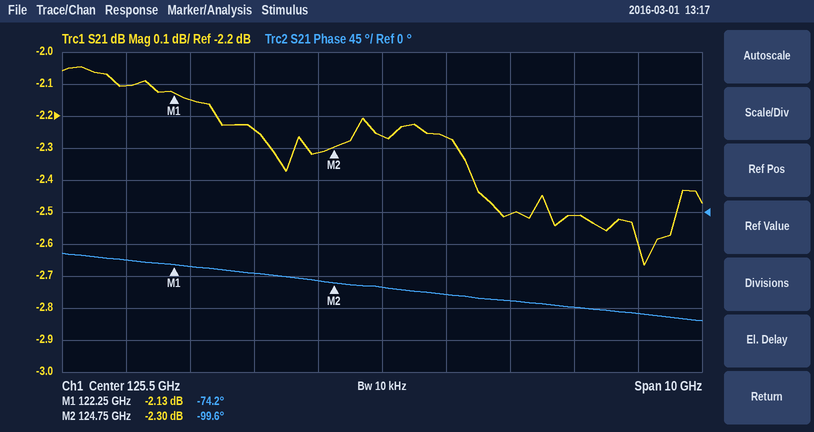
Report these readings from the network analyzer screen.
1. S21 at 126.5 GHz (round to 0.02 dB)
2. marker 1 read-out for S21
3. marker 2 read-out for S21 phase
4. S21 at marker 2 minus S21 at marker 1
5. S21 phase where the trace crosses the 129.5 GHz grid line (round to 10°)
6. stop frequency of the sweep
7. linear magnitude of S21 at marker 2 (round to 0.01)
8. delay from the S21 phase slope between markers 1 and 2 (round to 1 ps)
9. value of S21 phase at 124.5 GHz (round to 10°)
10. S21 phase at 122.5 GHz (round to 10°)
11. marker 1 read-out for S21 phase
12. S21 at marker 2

-2.26 dB
-2.13 dB
-99.6°
-0.17 dB
-140°
130.5 GHz
0.77
28 ps
-100°
-80°
-74.2°
-2.30 dB
